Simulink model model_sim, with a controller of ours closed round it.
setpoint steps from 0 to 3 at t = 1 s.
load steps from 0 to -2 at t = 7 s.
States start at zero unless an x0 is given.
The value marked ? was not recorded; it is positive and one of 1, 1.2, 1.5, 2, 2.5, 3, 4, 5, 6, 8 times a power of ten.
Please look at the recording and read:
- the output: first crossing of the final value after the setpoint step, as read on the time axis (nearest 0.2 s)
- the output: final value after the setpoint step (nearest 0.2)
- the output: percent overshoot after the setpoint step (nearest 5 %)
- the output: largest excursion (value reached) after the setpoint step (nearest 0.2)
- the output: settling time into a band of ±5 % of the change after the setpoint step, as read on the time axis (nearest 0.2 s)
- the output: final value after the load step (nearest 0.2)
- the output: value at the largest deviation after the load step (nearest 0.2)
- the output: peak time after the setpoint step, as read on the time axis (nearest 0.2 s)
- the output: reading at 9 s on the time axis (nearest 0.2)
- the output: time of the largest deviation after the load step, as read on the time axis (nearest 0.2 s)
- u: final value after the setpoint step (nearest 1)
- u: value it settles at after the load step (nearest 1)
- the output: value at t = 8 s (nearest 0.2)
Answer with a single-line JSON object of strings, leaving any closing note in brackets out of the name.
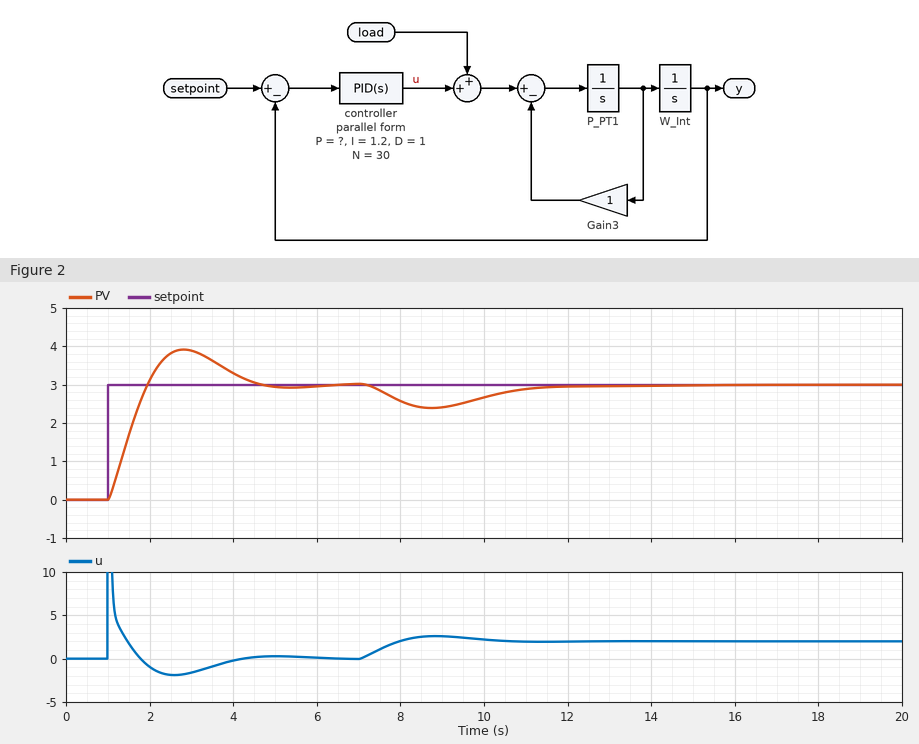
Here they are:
{"the output: first crossing of the final value after the setpoint step, as read on the time axis": "2.0 s", "the output: final value after the setpoint step": "3.0", "the output: percent overshoot after the setpoint step": "30 %", "the output: largest excursion (value reached) after the setpoint step": "4.0", "the output: settling time into a band of ±5 % of the change after the setpoint step, as read on the time axis": "4.2 s", "the output: final value after the load step": "3.0", "the output: value at the largest deviation after the load step": "2.4", "the output: peak time after the setpoint step, as read on the time axis": "2.8 s", "the output: reading at 9 s on the time axis": "2.4", "the output: time of the largest deviation after the load step, as read on the time axis": "8.8 s", "u: final value after the setpoint step": "0", "u: value it settles at after the load step": "2", "the output: value at t = 8 s": "2.6"}
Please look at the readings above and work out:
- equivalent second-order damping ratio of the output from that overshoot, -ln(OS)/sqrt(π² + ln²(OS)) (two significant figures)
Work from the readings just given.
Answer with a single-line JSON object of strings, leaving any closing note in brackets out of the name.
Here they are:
{"equivalent second-order damping ratio of the output from that overshoot, -ln(OS)/sqrt(π² + ln²(OS))": "0.36"}
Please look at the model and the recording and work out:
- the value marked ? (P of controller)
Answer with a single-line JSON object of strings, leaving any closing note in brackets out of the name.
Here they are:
{"the value marked ?": "3"}
